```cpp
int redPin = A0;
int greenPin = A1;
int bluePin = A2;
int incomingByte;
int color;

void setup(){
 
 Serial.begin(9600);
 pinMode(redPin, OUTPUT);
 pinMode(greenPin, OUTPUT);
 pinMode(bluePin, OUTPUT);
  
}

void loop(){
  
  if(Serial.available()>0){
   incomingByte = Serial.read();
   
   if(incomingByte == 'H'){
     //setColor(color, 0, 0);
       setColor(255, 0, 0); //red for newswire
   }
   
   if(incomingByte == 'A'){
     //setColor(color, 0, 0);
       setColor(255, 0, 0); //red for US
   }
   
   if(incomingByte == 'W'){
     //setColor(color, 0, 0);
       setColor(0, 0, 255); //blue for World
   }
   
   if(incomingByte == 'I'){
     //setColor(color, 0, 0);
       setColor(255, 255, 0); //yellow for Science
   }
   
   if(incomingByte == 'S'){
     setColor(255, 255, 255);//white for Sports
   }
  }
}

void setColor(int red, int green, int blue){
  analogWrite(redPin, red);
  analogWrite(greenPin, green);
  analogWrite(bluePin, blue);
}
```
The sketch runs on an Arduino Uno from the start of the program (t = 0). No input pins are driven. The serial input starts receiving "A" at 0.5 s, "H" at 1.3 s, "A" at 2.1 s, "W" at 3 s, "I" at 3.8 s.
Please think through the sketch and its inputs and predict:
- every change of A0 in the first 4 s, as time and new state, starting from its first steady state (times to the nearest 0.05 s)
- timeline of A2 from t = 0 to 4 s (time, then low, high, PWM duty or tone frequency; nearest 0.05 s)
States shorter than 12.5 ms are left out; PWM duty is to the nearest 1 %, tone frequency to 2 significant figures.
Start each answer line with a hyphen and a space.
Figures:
- 0 s low; 0.5 s high; 3 s low; 3.8 s high
- 0 s low; 3 s high; 3.8 s low
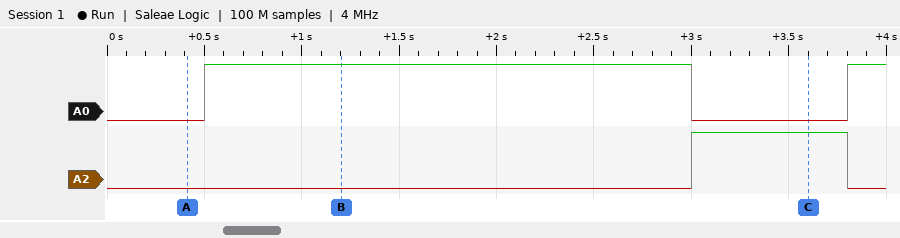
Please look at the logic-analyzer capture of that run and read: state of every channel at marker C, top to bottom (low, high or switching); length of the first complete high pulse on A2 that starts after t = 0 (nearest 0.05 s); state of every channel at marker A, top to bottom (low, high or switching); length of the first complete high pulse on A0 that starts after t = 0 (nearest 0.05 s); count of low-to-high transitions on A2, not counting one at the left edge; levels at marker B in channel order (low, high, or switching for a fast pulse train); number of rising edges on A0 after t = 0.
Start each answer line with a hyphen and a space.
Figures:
- A0 low, A2 high
- 0.80 s
- A0 low, A2 low
- 2.50 s
- 1
- A0 high, A2 low
- 2
